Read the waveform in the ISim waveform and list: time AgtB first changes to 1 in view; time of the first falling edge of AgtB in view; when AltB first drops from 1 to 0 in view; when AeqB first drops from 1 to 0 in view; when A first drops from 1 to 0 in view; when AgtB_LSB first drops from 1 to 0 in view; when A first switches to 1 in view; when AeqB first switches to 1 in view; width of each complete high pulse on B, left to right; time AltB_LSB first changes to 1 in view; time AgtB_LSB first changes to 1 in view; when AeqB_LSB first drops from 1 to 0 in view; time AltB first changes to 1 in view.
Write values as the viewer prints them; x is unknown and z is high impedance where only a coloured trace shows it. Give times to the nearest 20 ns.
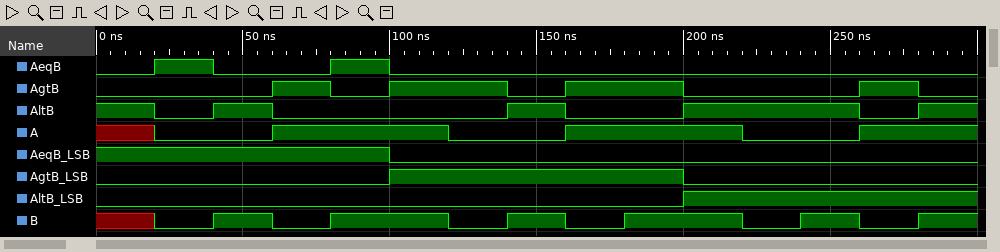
60 ns
80 ns
20 ns
40 ns
120 ns
200 ns
60 ns
20 ns
20 ns, 40 ns, 20 ns, 40 ns, 20 ns
200 ns
100 ns
100 ns
40 ns
